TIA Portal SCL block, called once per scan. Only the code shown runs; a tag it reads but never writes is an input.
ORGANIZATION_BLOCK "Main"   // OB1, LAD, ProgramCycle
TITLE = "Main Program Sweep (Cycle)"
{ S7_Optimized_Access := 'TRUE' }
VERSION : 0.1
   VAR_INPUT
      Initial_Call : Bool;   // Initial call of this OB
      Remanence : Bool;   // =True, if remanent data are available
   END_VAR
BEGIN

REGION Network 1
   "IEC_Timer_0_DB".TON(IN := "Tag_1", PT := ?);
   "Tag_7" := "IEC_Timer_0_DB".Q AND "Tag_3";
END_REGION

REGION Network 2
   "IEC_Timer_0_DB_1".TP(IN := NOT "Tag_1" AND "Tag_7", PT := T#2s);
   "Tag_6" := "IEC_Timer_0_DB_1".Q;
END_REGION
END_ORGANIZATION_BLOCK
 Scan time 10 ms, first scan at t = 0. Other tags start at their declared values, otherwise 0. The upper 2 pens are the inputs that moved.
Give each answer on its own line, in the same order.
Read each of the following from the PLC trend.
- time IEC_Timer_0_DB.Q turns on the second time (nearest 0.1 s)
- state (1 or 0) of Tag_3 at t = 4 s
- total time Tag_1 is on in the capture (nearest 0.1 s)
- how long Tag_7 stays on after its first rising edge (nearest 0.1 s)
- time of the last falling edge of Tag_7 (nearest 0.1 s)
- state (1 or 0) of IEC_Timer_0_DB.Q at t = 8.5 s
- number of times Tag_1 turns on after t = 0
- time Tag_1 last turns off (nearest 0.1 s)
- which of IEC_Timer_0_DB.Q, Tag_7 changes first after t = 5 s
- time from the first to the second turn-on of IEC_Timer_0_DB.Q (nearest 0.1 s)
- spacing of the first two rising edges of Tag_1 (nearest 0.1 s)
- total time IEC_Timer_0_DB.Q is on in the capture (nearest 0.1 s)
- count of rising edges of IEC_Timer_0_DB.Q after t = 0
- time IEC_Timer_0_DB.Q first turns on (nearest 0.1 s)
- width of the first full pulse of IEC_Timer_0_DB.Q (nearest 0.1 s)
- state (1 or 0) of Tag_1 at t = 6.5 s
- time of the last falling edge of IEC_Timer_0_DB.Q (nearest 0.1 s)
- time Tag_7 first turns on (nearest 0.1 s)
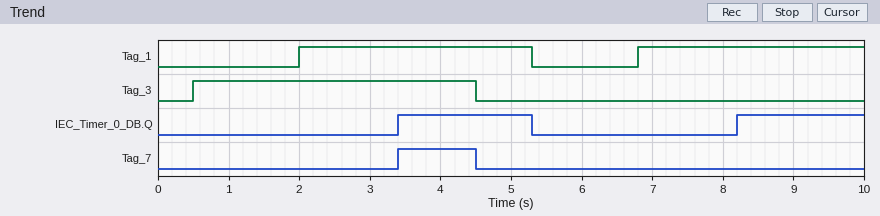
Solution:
8.2 s
1
6.5 s
1.1 s
4.5 s
1
2
5.3 s
IEC_Timer_0_DB.Q
4.8 s
4.8 s
3.7 s
2
3.4 s
1.9 s
0
5.3 s
3.4 s
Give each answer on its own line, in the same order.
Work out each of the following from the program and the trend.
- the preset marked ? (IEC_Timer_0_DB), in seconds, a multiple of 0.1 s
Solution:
1.4 s
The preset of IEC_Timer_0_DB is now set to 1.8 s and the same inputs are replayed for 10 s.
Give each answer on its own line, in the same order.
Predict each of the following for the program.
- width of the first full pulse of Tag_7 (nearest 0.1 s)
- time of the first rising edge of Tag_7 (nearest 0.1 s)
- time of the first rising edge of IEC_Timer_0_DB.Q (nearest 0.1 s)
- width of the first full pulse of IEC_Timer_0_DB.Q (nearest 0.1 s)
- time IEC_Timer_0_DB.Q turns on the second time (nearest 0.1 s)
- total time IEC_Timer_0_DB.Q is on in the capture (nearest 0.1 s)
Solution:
0.7 s
3.8 s
3.8 s
1.5 s
8.6 s
2.9 s
